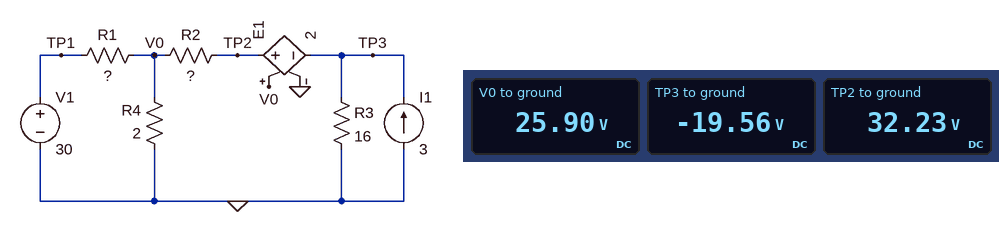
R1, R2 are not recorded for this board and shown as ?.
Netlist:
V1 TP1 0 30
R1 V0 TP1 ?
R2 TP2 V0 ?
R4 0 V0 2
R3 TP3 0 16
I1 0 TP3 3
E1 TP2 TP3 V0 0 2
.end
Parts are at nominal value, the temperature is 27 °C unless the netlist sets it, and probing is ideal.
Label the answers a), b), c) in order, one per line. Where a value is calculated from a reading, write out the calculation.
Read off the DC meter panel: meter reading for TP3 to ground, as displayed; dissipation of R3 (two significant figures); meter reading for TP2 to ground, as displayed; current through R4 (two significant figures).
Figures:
a) -19.56 V
b) (0 V - (-19.56 V))^2 / 16 Ω = 24 W
c) 32.23 V
d) (25.9 V) / 2 Ω = 13 A
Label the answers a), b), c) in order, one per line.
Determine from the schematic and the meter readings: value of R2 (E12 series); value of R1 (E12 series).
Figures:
a) 1.5 Ω
b) 0.47 Ω
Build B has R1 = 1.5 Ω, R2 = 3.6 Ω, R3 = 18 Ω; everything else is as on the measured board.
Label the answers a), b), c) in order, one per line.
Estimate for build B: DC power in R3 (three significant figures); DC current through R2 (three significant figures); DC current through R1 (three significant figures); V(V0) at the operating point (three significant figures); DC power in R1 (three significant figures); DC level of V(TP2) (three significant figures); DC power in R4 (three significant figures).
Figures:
a) 3.32 W
b) 3.43 A
c) 6.61 A
d) 20.1 V
e) 65.6 W
f) 32.4 V
g) 202 W
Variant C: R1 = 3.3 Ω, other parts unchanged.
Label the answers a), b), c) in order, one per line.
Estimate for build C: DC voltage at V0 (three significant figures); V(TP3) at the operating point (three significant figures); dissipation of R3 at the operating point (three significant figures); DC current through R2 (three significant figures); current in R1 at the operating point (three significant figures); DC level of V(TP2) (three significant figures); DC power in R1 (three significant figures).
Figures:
a) 15.9 V
b) -10.4 V
c) 6.75 W
d) 3.65 A
e) 4.28 A
f) 21.3 V
g) 60.5 W
